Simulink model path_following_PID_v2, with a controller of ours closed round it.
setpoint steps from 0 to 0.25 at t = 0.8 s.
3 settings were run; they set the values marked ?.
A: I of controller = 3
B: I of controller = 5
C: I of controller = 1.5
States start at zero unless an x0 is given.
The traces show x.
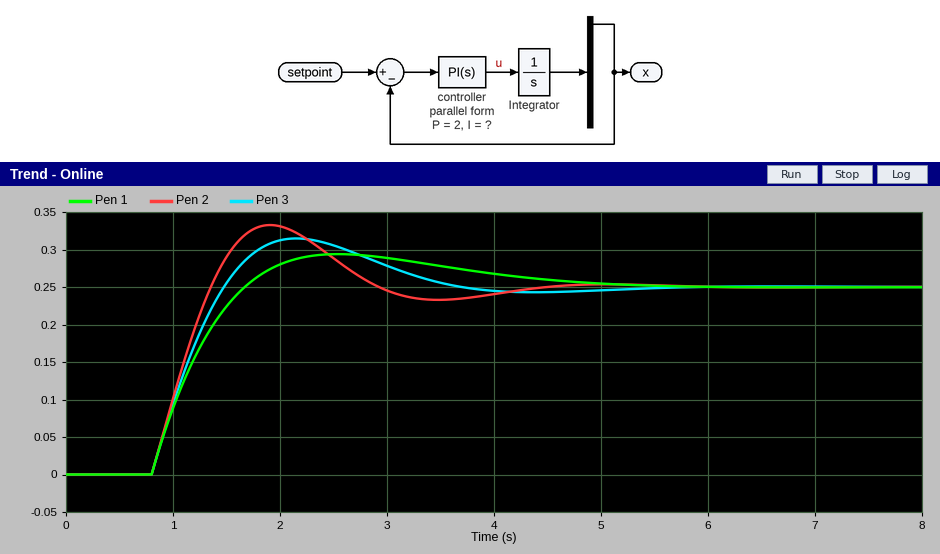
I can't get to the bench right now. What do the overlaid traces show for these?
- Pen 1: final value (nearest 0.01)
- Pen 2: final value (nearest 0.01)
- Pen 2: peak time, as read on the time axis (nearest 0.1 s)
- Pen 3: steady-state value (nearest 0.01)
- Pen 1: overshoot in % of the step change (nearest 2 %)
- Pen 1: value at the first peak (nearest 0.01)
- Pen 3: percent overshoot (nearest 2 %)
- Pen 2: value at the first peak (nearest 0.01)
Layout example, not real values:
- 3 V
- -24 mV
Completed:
- 0.25
- 0.25
- 1.9 s
- 0.25
- 18 %
- 0.29
- 26 %
- 0.33
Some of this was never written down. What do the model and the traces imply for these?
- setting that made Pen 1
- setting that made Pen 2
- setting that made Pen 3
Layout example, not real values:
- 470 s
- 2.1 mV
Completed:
- C
- B
- A
